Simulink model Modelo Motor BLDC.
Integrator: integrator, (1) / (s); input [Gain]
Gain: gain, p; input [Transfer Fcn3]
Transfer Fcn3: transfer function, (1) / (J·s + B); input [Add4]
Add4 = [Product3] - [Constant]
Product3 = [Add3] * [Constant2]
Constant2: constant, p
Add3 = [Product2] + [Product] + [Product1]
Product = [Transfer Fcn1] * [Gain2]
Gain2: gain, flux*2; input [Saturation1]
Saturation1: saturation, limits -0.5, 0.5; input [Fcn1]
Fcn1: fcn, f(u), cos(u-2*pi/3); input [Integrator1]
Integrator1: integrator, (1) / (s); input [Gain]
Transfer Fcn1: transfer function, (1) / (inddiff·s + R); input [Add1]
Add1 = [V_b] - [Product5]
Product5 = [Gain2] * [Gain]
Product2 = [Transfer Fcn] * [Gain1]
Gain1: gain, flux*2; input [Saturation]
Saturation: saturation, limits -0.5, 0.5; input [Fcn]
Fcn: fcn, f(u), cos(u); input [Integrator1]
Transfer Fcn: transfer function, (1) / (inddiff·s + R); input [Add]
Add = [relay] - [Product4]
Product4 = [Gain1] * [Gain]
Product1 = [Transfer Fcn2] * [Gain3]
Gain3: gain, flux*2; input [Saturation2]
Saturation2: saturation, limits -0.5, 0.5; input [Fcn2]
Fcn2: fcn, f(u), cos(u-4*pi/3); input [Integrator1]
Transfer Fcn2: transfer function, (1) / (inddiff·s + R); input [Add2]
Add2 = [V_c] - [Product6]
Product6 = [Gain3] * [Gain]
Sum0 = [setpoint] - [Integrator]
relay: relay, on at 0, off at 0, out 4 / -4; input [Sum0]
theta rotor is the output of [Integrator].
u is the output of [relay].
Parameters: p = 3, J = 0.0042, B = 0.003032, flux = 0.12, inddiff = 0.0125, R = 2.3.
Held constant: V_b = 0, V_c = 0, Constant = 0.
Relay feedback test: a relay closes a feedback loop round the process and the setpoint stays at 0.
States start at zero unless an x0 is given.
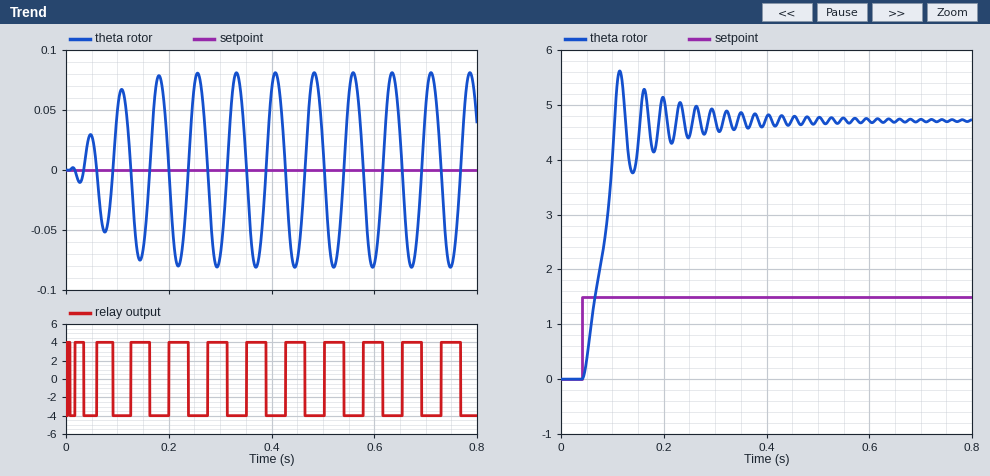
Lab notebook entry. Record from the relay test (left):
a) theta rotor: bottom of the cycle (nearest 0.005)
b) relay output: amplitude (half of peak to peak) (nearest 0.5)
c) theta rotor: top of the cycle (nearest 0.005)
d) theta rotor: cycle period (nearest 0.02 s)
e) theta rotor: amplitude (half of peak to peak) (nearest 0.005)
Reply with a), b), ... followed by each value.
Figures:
a) -0.080
b) 4.0
c) 0.080
d) 0.08 s
e) 0.080
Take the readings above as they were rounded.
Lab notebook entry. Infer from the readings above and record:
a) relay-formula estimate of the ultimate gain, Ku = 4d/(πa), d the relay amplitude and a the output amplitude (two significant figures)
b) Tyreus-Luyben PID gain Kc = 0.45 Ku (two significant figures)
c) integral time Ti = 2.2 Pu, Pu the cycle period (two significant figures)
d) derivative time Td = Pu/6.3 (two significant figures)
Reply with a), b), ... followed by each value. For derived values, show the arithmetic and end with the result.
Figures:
a) 4 × 4 / (π × 0.08) = 64
b) 0.45 × 64 = 29
c) 2.2 × 0.08 = 0.18 s
d) 0.08 / 6.3 = 0.013 s
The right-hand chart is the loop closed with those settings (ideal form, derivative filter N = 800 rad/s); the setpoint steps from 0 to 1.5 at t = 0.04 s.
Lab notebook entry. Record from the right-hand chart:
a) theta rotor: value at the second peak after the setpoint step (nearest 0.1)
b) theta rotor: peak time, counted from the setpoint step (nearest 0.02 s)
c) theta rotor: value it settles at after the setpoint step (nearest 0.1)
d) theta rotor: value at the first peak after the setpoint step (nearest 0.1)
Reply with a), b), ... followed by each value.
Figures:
a) 5.3
b) 0.08 s
c) 4.7
d) 5.6
